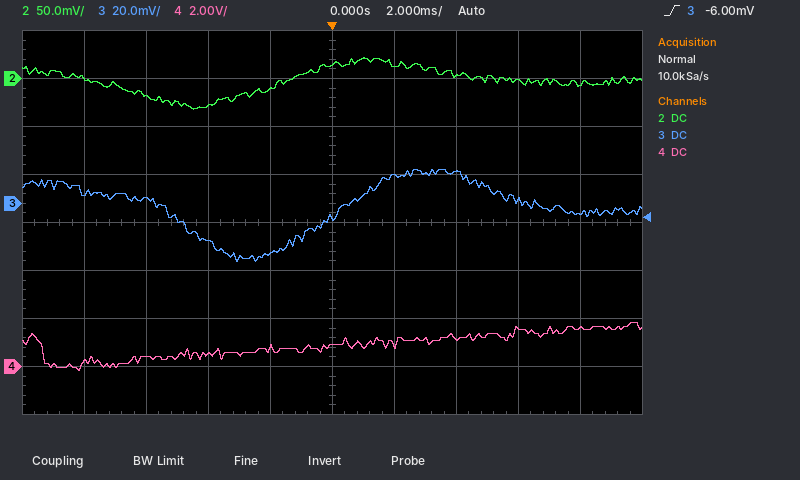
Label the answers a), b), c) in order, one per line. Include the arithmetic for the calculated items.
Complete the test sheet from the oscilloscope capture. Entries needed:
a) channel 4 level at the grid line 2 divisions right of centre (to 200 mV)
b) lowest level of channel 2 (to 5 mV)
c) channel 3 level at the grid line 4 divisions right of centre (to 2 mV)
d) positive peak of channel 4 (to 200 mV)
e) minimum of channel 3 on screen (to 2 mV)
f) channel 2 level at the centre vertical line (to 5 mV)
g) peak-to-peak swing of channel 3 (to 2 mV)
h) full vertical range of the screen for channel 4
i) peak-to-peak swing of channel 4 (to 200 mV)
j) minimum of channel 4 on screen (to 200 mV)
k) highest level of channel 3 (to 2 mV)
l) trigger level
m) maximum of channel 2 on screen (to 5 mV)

a) 1.2 V
b) -30 mV
c) -4 mV
d) 1.8 V
e) -24 mV
f) 15 mV
g) 14 mV − (-24 mV) = 38 mV
h) 16 V
i) 1.8 V − (-200 mV) = 2.0 V
j) -200 mV
k) 14 mV
l) -6.00 mV
m) 20 mV
